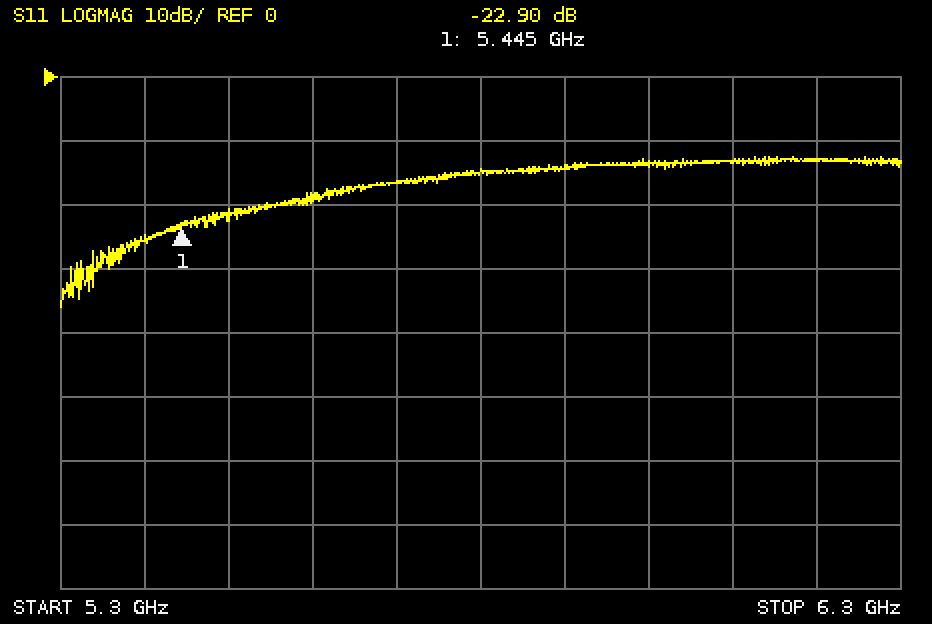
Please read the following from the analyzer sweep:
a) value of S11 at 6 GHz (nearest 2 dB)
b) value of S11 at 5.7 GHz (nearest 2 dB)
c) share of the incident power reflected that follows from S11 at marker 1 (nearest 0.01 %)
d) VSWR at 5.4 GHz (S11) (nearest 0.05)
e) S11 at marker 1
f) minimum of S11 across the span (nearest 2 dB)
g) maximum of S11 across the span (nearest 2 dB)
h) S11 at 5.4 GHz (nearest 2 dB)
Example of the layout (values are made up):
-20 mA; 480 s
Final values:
-14 dB; -16 dB; 0.51 %; 1.10; -22.90 dB; -36 dB; -12 dB; -26 dB
